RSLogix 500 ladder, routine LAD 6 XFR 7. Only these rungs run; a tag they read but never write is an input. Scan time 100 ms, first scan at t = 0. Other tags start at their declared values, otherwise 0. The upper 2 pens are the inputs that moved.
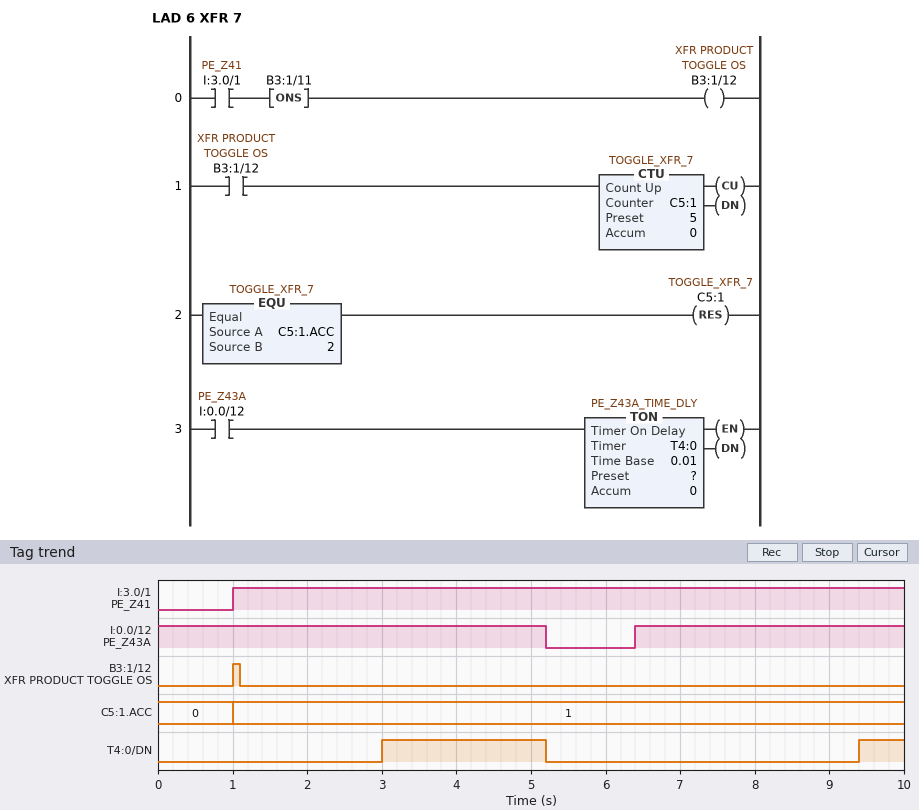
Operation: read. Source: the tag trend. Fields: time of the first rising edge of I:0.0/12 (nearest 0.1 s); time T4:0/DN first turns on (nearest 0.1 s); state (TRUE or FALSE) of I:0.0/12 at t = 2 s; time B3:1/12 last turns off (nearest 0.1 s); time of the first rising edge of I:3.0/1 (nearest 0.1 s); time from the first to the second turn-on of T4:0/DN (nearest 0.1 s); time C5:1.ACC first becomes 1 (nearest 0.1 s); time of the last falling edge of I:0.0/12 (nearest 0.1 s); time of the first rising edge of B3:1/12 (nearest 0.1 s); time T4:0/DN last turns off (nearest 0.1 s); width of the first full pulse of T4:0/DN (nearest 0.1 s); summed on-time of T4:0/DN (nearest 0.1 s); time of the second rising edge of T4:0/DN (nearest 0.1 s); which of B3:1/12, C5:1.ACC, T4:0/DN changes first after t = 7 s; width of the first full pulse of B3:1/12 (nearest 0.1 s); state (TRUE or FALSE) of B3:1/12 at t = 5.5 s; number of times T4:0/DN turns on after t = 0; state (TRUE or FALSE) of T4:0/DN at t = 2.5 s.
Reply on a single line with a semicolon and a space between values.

6.4 s; 3.0 s; TRUE; 1.1 s; 1.0 s; 6.4 s; 1.0 s; 5.2 s; 1.0 s; 5.2 s; 2.2 s; 2.8 s; 9.4 s; T4:0/DN; 0.1 s; FALSE; 2; FALSE
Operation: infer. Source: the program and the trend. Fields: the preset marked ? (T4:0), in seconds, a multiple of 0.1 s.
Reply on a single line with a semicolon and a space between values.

3.0 s
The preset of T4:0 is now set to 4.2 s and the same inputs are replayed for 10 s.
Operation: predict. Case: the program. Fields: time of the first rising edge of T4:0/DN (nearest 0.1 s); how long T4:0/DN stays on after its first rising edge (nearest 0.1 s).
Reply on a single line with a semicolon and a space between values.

4.2 s; 1.0 s
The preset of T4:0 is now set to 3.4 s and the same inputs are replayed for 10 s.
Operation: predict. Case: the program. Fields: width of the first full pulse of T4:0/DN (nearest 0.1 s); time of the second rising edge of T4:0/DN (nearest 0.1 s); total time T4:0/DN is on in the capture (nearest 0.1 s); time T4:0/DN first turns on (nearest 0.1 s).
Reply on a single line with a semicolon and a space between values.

1.8 s; 9.8 s; 2.0 s; 3.4 s
